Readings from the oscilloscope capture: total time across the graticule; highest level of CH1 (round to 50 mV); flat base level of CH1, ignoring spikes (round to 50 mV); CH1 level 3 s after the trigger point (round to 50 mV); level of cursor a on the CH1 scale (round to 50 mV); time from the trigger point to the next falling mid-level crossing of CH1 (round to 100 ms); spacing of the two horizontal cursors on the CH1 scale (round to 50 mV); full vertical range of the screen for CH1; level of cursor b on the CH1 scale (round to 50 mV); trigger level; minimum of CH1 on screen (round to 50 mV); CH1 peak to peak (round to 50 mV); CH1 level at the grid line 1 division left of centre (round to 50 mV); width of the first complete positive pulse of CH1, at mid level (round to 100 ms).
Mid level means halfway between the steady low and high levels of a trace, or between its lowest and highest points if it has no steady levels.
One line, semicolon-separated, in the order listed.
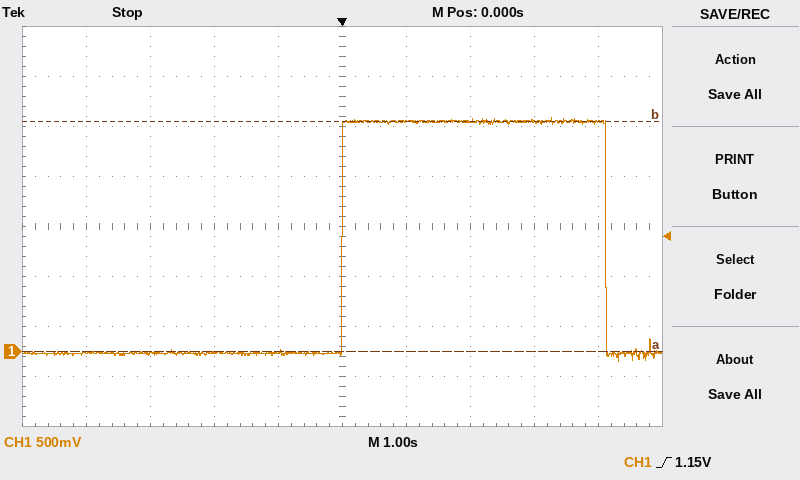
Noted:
10 s; 2.35 V; 0 mV; 2.30 V; 0 mV; 4.1 s; 2.30 V; 4 V; 2.30 V; 1.15 V; -100 mV; 2.45 V; 0 mV; 4.1 s
